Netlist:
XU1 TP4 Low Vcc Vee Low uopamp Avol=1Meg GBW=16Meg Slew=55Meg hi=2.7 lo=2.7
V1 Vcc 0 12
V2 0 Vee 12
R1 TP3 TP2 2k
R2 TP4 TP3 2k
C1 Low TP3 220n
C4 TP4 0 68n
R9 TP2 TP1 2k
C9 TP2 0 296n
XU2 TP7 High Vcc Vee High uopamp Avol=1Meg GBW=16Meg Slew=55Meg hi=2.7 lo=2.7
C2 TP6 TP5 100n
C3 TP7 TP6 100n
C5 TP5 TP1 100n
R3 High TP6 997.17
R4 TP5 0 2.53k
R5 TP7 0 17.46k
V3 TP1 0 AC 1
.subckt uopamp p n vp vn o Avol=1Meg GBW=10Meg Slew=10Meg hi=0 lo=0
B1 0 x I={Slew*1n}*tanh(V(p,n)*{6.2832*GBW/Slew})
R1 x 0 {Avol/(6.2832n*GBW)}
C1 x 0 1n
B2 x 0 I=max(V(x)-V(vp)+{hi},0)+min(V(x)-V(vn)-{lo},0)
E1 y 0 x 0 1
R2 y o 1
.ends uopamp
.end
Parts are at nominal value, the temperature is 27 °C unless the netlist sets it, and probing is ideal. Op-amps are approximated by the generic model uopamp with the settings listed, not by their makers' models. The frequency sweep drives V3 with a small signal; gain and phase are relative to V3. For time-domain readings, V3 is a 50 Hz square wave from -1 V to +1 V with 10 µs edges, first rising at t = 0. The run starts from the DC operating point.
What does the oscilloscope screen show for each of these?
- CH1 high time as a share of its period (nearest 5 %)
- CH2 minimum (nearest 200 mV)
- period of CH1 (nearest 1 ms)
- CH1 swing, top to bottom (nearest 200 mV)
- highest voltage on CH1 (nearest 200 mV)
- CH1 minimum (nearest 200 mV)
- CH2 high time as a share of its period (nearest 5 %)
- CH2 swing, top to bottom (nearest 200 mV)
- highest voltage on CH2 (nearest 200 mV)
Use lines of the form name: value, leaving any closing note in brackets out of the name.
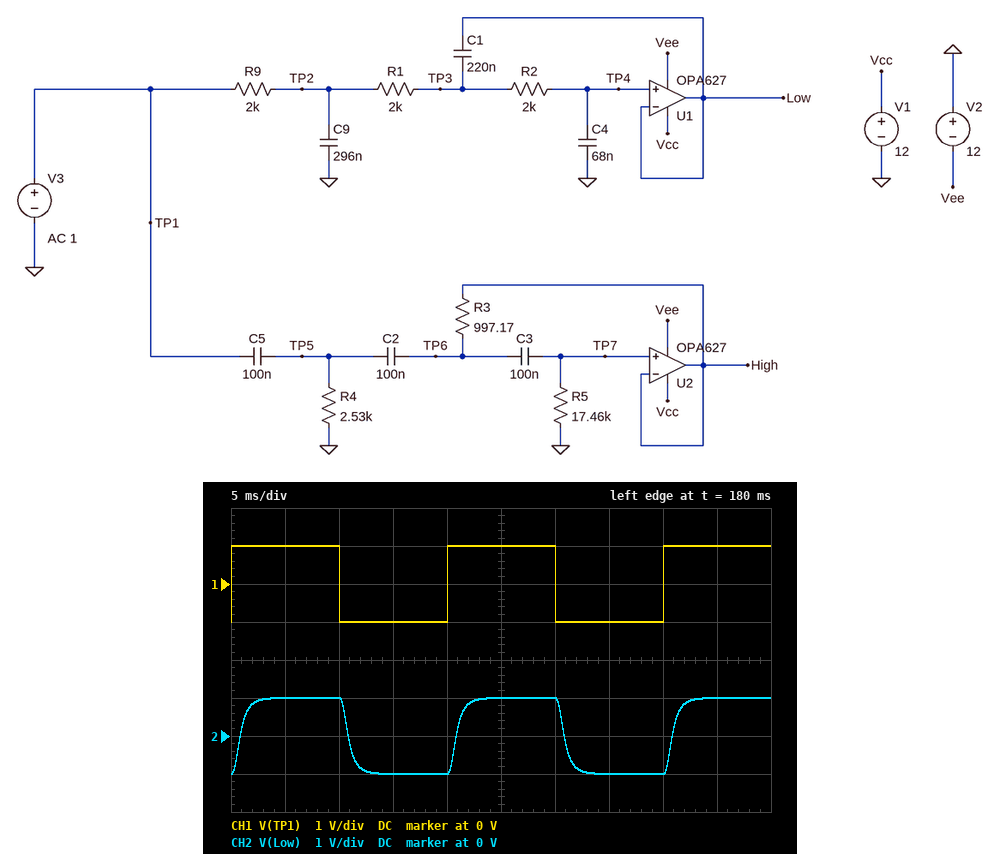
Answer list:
CH1 high time as a share of its period: 50 %
CH2 minimum: -1.0 V
period of CH1: 20 ms
CH1 swing, top to bottom: 2.0 V
highest voltage on CH1: 1.0 V
CH1 minimum: -1.0 V
CH2 high time as a share of its period: 50 %
CH2 swing, top to bottom: 2.0 V
highest voltage on CH2: 1.0 V
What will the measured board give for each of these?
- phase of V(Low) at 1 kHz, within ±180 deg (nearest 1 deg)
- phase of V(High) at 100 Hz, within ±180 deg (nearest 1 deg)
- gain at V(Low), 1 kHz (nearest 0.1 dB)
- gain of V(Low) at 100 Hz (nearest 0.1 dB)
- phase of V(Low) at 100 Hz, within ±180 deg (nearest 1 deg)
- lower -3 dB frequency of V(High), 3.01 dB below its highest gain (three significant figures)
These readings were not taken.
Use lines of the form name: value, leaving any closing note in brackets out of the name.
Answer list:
phase of V(Low) at 1 kHz, within ±180 deg: 166 deg
phase of V(High) at 100 Hz, within ±180 deg: -116 deg
gain at V(Low), 1 kHz: -20.3 dB
gain of V(Low) at 100 Hz: -0.7 dB
phase of V(Low) at 100 Hz, within ±180 deg: -35 deg
lower -3 dB frequency of V(High), 3.01 dB below its highest gain: 451 Hz
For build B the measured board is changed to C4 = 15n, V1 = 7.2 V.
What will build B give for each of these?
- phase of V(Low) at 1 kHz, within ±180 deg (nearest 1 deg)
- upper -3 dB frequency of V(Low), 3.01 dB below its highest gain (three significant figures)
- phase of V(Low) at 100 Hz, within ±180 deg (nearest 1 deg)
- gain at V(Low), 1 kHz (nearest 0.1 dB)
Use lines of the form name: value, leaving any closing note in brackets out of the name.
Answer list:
phase of V(Low) at 1 kHz, within ±180 deg: -122 deg
upper -3 dB frequency of V(Low), 3.01 dB below its highest gain: 281 Hz
phase of V(Low) at 100 Hz, within ±180 deg: -24 deg
gain at V(Low), 1 kHz: -8.8 dB
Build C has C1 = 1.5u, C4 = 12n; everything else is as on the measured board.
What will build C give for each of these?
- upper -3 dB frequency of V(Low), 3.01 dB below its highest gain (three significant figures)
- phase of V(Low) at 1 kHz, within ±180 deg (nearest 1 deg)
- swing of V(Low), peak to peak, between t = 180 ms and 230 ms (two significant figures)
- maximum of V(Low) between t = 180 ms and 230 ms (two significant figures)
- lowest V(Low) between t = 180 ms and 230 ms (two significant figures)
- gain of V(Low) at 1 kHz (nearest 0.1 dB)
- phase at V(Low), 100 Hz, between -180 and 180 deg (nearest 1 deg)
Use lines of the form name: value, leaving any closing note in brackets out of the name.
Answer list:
upper -3 dB frequency of V(Low), 3.01 dB below its highest gain: 589 Hz
phase of V(Low) at 1 kHz, within ±180 deg: 132 deg
swing of V(Low), peak to peak, between t = 180 ms and 230 ms: 2.4 V
maximum of V(Low) between t = 180 ms and 230 ms: 1.2 V
lowest V(Low) between t = 180 ms and 230 ms: -1.2 V
gain of V(Low) at 1 kHz: -18.7 dB
phase at V(Low), 100 Hz, between -180 and 180 deg: -24 deg
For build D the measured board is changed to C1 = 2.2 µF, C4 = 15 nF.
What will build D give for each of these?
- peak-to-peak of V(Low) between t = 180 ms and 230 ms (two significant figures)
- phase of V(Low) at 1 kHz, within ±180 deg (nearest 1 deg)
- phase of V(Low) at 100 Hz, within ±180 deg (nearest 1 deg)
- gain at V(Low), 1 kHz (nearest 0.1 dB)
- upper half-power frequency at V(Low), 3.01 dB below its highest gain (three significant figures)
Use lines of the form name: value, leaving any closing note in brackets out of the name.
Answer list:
peak-to-peak of V(Low) between t = 180 ms and 230 ms: 2.9 V
phase of V(Low) at 1 kHz, within ±180 deg: 126 deg
phase of V(Low) at 100 Hz, within ±180 deg: -25 deg
gain at V(Low), 1 kHz: -25.4 dB
upper half-power frequency at V(Low), 3.01 dB below its highest gain: 411 Hz
